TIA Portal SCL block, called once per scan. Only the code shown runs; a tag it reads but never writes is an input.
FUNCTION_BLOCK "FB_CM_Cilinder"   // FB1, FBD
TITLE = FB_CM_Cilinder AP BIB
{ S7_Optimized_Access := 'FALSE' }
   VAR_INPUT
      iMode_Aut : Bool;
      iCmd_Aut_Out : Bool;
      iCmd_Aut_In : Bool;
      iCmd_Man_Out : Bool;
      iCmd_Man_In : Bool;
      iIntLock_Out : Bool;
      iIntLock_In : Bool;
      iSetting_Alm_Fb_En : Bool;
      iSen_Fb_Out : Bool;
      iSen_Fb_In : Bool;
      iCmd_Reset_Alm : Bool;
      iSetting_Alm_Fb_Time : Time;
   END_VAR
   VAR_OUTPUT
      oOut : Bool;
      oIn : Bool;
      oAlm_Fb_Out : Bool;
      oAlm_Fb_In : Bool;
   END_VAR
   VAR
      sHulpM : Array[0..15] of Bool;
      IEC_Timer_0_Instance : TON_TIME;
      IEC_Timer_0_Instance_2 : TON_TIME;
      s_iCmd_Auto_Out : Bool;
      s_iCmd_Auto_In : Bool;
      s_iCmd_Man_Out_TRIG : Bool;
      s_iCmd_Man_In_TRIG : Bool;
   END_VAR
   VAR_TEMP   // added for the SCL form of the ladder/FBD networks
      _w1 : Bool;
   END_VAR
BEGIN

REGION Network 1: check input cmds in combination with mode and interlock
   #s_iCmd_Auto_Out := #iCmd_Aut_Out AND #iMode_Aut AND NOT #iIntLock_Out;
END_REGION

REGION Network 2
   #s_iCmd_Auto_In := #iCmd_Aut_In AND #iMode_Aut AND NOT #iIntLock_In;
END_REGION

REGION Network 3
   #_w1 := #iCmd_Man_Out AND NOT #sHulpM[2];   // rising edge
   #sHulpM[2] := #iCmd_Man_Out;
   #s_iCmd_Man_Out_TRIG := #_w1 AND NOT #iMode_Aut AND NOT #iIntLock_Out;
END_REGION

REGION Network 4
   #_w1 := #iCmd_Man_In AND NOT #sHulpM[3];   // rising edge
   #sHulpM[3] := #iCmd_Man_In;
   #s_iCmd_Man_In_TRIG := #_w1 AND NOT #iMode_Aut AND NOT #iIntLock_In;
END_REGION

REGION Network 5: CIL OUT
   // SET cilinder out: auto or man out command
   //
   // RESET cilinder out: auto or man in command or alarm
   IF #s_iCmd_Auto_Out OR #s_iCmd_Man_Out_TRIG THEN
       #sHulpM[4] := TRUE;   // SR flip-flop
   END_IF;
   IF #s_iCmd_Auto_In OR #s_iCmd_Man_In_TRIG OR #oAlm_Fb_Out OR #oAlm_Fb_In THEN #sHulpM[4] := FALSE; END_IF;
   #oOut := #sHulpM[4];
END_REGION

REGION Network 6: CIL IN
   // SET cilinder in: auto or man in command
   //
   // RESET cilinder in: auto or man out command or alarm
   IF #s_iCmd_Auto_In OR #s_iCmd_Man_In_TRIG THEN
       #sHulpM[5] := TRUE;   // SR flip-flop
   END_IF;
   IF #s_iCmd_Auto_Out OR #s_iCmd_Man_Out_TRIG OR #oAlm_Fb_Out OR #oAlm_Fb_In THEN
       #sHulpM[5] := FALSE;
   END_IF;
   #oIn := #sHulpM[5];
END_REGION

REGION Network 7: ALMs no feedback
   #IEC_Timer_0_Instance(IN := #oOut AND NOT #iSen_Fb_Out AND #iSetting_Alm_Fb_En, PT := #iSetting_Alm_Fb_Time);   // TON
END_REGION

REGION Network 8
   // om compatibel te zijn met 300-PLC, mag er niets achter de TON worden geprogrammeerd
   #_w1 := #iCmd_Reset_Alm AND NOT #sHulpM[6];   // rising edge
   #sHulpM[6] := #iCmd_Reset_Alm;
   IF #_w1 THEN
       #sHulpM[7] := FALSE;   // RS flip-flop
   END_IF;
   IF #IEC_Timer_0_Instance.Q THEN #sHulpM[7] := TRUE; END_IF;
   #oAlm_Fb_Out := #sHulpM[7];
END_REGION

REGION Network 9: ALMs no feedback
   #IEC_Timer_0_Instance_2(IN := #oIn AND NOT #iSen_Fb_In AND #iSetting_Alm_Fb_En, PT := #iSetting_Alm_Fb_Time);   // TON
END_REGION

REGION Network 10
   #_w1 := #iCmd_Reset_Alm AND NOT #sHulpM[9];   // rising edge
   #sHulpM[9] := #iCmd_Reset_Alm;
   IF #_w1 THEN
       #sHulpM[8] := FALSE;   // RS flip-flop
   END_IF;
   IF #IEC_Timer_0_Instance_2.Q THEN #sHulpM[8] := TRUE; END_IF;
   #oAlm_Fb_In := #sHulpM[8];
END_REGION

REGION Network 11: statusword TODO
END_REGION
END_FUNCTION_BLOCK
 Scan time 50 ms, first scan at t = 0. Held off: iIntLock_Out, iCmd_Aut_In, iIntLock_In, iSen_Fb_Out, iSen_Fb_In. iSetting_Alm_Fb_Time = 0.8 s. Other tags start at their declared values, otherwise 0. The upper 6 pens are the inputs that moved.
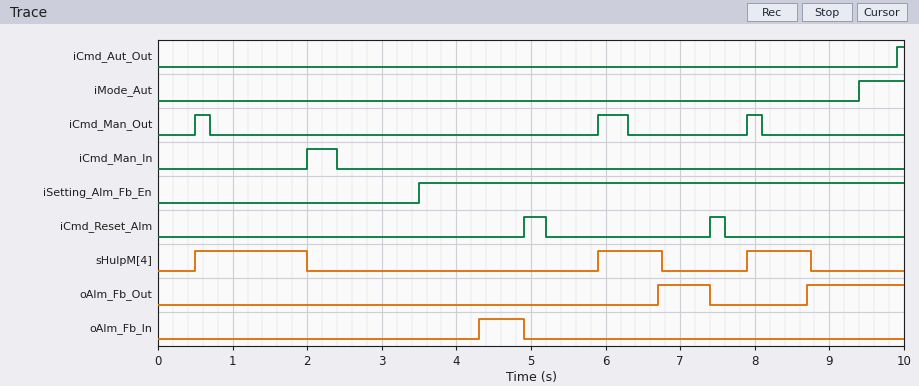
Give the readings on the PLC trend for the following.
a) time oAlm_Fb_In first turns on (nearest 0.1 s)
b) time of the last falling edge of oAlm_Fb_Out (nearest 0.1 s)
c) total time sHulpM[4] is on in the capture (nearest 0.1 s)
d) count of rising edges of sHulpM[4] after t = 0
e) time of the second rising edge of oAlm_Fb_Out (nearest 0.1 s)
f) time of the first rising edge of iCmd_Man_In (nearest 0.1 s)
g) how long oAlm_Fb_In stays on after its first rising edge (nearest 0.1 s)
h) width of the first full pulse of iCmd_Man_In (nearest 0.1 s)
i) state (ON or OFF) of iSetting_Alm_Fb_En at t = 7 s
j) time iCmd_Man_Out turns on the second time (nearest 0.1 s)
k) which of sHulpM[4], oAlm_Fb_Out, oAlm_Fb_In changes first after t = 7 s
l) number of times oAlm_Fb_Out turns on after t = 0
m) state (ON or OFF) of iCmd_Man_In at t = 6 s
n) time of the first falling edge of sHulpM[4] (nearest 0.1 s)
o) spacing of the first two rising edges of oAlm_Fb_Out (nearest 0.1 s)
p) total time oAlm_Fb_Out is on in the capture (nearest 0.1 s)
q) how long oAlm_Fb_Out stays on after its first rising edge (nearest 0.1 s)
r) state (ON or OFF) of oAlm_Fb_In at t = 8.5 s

4.3 s
7.4 s
3.2 s
3
8.7 s
2.0 s
0.6 s
0.4 s
ON
5.9 s
oAlm_Fb_Out
2
OFF
2.0 s
2.0 s
2.0 s
0.7 s
OFF
